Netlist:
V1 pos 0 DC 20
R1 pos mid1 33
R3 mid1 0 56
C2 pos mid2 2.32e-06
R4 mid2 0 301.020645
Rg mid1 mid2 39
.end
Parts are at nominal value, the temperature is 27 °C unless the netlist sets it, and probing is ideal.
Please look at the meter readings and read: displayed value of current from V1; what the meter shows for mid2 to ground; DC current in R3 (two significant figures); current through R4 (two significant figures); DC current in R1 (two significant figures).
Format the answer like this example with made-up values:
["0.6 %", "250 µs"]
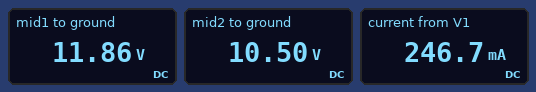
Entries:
["246.7 mA", "10.50 V", "210 mA", "35 mA", "250 mA"]
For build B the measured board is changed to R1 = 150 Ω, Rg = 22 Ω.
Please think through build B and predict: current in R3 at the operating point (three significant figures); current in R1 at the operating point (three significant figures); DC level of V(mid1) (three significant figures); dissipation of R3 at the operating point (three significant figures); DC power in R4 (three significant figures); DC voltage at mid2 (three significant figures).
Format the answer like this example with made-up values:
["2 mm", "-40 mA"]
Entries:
["86.2 mA", "101 mA", "4.83 V", "416 mW", "67.2 mW", "4.50 V"]
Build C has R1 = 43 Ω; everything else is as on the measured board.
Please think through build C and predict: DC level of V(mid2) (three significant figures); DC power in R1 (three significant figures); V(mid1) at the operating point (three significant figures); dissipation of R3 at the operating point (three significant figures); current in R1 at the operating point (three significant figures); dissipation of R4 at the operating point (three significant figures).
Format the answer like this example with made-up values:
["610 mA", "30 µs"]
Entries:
["9.35 V", "2.07 W", "10.6 V", "1.99 W", "220 mA", "290 mW"]
